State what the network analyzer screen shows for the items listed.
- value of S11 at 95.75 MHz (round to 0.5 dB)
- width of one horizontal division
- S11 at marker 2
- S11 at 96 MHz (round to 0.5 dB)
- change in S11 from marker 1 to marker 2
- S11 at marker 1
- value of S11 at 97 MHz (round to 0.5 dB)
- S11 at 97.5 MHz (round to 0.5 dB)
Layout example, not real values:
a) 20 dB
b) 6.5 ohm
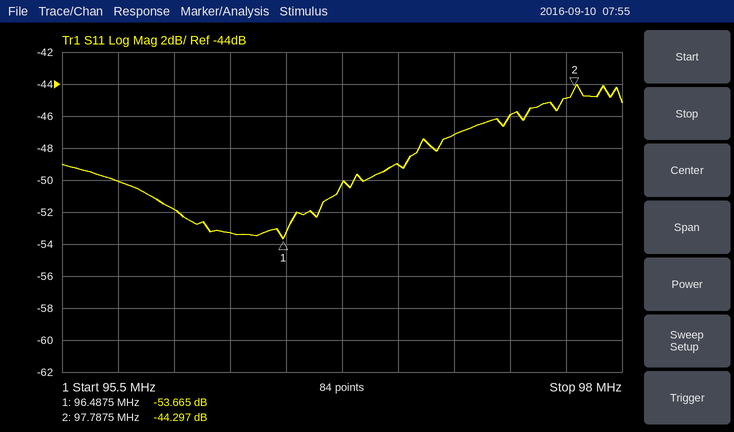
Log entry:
a) -50.0 dB
b) 250 kHz
c) -44.297 dB
d) -52.0 dB
e) 9.368 dB
f) -53.665 dB
g) -49.0 dB
h) -46.0 dB
